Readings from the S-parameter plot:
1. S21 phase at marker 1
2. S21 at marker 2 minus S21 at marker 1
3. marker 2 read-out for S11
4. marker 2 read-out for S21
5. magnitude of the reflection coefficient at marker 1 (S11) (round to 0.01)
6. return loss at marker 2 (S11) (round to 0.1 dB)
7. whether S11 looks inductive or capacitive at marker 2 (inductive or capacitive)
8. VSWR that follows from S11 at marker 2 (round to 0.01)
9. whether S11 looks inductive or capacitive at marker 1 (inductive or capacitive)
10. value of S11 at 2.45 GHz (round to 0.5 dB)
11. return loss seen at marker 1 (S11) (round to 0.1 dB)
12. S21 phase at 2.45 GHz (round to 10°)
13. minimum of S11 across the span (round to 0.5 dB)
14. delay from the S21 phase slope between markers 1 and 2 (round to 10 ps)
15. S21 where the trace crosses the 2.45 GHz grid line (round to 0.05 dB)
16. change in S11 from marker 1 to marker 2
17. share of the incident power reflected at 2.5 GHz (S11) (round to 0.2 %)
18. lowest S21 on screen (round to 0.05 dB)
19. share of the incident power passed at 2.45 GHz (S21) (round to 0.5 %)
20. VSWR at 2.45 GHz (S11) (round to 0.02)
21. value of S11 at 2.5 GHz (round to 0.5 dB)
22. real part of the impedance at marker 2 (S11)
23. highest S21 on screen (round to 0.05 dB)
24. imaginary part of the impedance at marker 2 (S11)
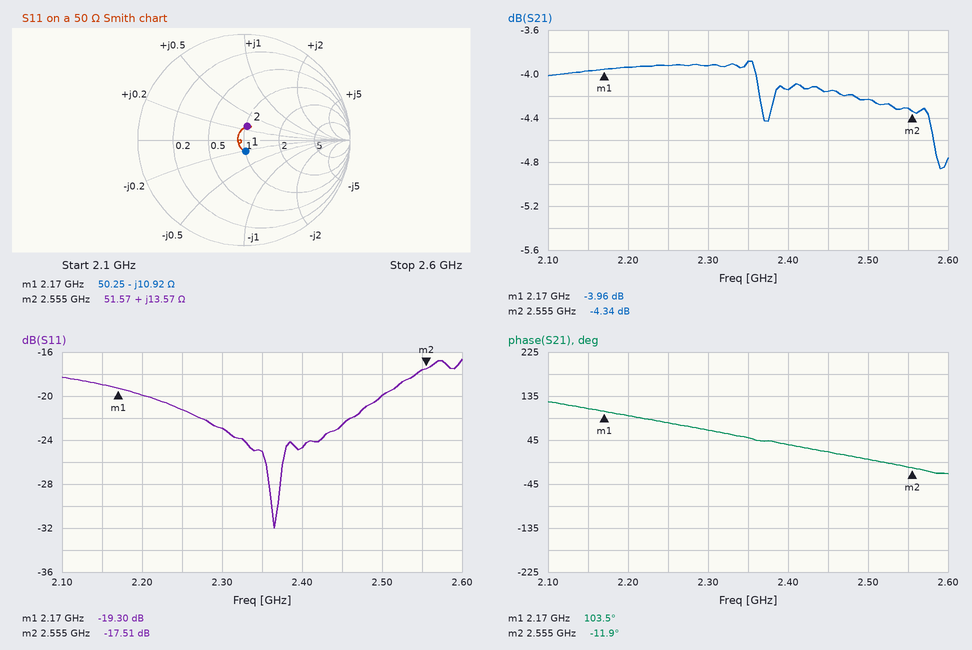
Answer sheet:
103.5°
-0.38 dB
-17.51 dB
-4.34 dB
0.11
17.5 dB
inductive
1.31
capacitive
-22.5 dB
19.3 dB
20°
-32.0 dB
830 ps
-4.15 dB
1.79 dB
1.0 %
-4.85 dB
38.5 %
1.16
-20.0 dB
51.57 Ω
-3.90 dB
+13.57 Ω
